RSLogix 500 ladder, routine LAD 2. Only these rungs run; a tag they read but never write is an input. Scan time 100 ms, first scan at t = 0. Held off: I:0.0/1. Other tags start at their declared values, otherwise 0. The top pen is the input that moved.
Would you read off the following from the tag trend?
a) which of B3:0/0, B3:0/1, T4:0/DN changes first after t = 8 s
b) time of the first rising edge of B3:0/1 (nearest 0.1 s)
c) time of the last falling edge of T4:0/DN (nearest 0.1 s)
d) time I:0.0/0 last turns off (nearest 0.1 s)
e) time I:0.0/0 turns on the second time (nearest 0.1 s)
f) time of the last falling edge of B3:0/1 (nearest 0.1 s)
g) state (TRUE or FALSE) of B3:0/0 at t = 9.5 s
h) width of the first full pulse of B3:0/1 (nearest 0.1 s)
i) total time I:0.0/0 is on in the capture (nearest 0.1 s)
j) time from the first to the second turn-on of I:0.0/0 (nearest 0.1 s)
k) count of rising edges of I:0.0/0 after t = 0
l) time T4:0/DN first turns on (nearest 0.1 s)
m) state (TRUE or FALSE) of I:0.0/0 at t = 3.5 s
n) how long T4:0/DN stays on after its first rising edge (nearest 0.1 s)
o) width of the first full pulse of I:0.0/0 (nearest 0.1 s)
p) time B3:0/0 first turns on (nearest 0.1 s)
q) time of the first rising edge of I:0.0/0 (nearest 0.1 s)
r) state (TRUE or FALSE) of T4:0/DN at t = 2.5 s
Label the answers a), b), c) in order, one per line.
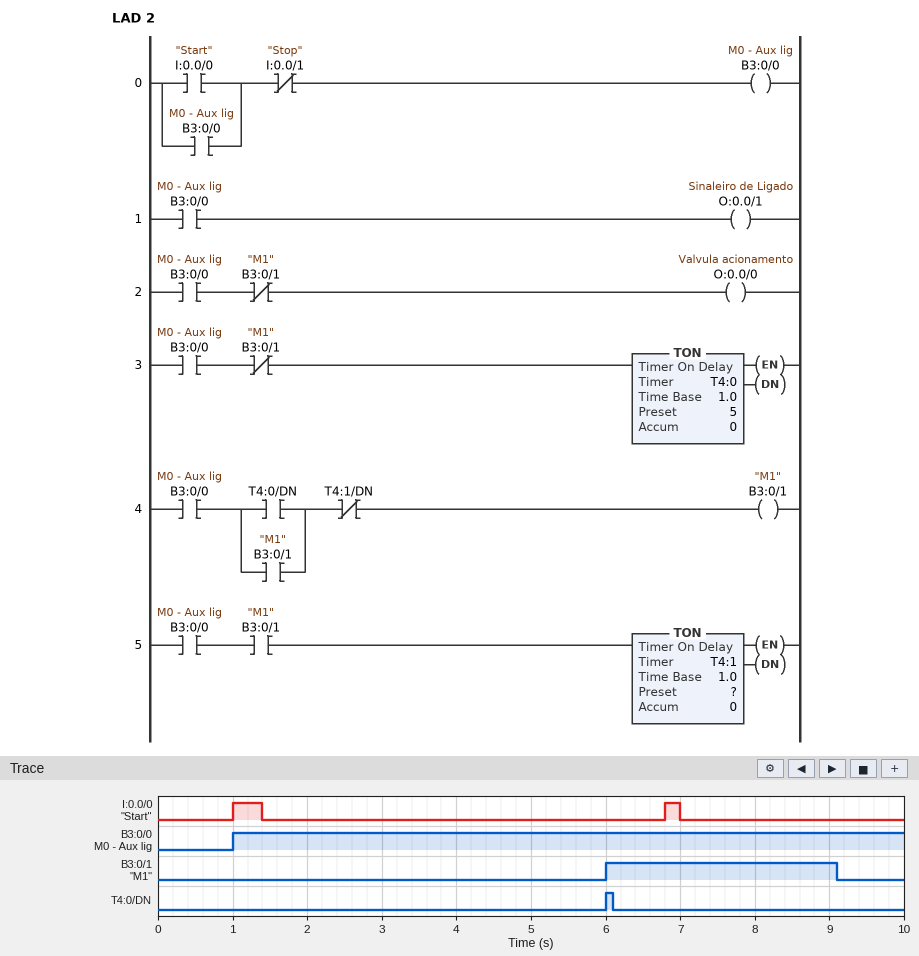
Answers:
a) B3:0/1
b) 6.0 s
c) 6.1 s
d) 7.0 s
e) 6.8 s
f) 9.1 s
g) TRUE
h) 3.1 s
i) 0.6 s
j) 5.8 s
k) 2
l) 6.0 s
m) FALSE
n) 0.1 s
o) 0.4 s
p) 1.0 s
q) 1.0 s
r) FALSE
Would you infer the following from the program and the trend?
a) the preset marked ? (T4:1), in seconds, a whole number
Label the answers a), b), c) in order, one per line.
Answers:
a) 3 s
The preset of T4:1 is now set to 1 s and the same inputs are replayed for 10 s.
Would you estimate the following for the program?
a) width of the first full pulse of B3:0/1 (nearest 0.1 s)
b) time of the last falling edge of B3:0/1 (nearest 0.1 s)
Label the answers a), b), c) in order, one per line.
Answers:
a) 1.1 s
b) 7.1 s
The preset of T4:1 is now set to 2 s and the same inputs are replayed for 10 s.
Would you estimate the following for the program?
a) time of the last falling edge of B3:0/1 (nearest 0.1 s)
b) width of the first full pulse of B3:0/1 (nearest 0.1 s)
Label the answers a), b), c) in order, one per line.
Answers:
a) 8.1 s
b) 2.1 s
